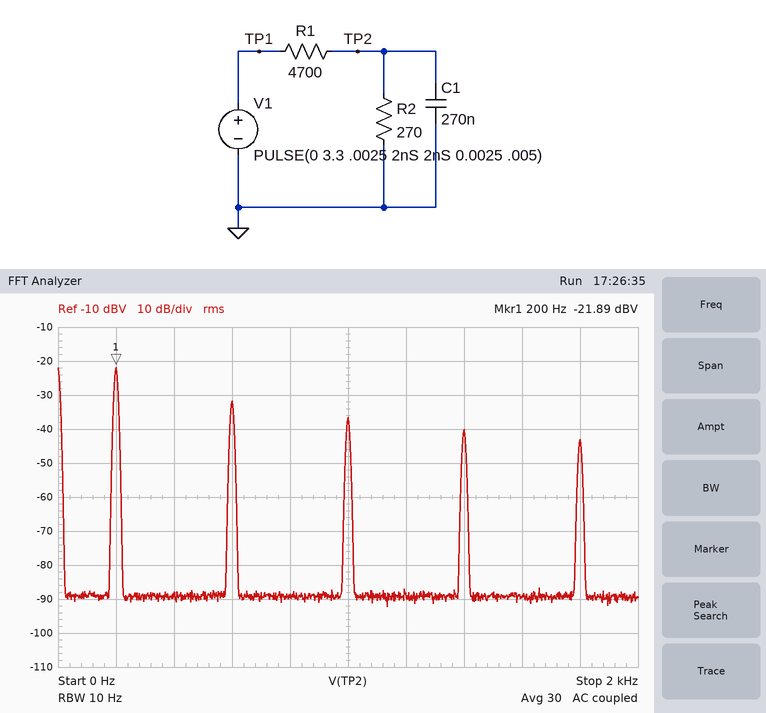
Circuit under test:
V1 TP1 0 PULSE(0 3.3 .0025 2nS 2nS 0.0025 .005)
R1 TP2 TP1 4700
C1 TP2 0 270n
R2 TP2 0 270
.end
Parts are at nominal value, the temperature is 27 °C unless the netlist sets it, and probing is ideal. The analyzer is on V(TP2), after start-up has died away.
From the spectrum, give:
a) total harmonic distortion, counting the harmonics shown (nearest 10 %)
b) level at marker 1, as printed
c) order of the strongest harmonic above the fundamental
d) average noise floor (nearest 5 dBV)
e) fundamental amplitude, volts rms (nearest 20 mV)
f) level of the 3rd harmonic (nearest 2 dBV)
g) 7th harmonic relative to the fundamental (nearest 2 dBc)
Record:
40 %
-21.89 dBV
3
-90 dBV
80 mV
-32 dBV
-18 dBc
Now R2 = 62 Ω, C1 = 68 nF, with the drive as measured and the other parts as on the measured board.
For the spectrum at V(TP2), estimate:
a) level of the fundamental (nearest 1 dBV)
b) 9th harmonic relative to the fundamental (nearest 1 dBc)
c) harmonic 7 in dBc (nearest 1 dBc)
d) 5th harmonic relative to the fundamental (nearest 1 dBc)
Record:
-34 dBV
-19 dBc
-17 dBc
-14 dBc
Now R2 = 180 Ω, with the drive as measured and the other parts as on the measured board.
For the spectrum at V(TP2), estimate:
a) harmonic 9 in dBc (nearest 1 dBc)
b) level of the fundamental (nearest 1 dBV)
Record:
-20 dBc
-25 dBV
